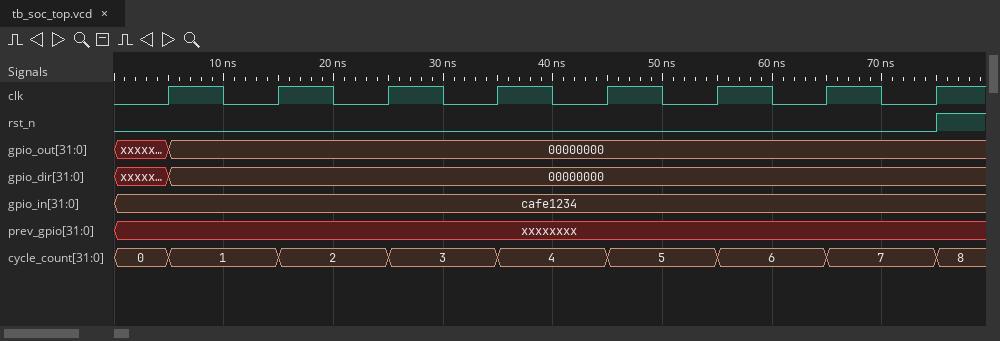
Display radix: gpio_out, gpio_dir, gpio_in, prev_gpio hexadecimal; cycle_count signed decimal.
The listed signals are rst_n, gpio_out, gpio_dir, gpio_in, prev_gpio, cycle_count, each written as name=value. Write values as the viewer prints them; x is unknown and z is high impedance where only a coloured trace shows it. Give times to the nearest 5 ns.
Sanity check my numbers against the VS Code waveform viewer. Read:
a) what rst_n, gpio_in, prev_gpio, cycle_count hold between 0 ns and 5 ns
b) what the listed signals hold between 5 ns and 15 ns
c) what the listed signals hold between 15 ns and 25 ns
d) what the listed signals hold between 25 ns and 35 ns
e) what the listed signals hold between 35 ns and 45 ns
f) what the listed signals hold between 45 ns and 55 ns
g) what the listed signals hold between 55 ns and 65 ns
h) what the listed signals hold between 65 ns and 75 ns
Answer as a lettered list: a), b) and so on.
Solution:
a) rst_n=0, gpio_in=cafe1234, prev_gpio=xxxxxxxx, cycle_count=0
b) rst_n=0, gpio_out=00000000, gpio_dir=00000000, gpio_in=cafe1234, prev_gpio=xxxxxxxx, cycle_count=1
c) rst_n=0, gpio_out=00000000, gpio_dir=00000000, gpio_in=cafe1234, prev_gpio=xxxxxxxx, cycle_count=2
d) rst_n=0, gpio_out=00000000, gpio_dir=00000000, gpio_in=cafe1234, prev_gpio=xxxxxxxx, cycle_count=3
e) rst_n=0, gpio_out=00000000, gpio_dir=00000000, gpio_in=cafe1234, prev_gpio=xxxxxxxx, cycle_count=4
f) rst_n=0, gpio_out=00000000, gpio_dir=00000000, gpio_in=cafe1234, prev_gpio=xxxxxxxx, cycle_count=5
g) rst_n=0, gpio_out=00000000, gpio_dir=00000000, gpio_in=cafe1234, prev_gpio=xxxxxxxx, cycle_count=6
h) rst_n=0, gpio_out=00000000, gpio_dir=00000000, gpio_in=cafe1234, prev_gpio=xxxxxxxx, cycle_count=7
